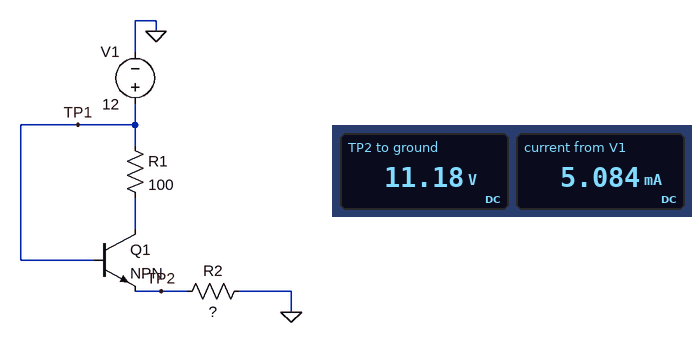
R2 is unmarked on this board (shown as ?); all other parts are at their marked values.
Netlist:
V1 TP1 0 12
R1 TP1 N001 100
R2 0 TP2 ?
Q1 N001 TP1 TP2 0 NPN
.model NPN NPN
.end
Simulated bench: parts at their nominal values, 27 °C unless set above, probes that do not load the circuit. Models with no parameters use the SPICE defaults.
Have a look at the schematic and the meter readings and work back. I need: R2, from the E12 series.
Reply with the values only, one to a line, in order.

2.2 kΩ
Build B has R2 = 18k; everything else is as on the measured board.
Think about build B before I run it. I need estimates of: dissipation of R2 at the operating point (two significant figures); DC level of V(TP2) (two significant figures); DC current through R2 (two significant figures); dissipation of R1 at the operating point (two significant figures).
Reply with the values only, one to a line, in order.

7.0 mW
11 V
620 µA
38 µW
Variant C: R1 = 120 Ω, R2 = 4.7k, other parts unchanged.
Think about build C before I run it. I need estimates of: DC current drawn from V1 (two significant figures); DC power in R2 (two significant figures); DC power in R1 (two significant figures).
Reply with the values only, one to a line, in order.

2.4 mA
27 mW
670 µW
